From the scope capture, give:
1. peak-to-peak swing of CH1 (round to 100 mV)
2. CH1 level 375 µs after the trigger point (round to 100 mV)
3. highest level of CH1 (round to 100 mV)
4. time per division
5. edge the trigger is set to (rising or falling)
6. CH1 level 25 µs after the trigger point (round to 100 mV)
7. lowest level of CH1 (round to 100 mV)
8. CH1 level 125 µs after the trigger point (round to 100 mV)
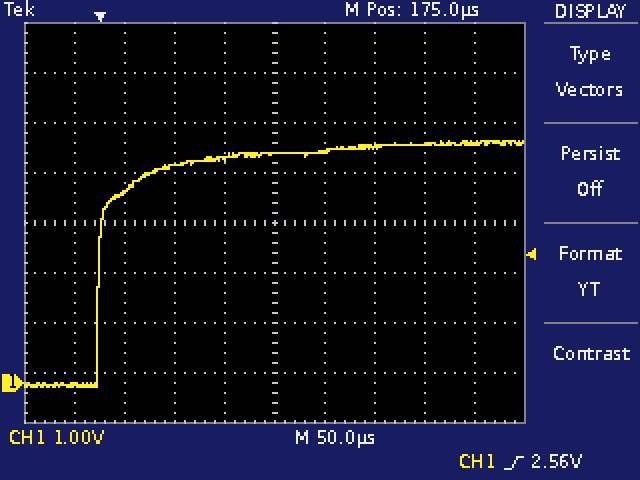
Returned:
4.9 V
4.8 V
4.8 V
50 µs
rising
3.8 V
-100 mV
4.5 V
